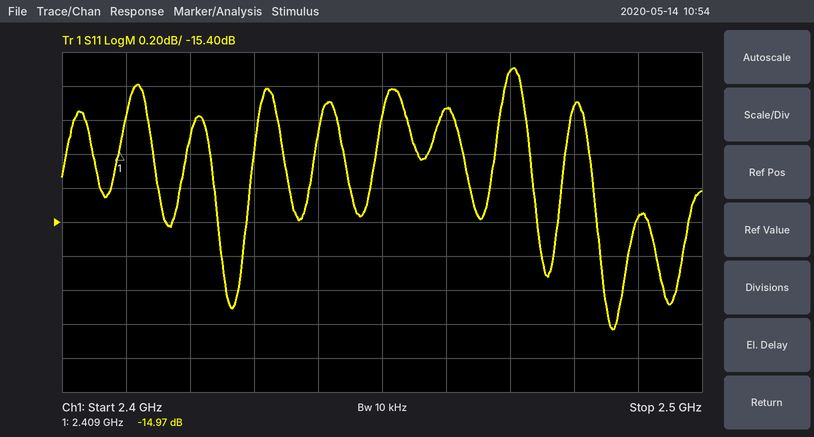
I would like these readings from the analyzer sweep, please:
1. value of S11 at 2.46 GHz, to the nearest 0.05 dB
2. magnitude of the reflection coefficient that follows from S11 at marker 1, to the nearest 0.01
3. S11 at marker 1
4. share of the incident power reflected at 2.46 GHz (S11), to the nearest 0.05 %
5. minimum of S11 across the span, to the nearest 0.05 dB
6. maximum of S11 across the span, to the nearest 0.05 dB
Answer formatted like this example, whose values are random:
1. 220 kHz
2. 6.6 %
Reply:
1. -14.75 dB
2. 0.18
3. -14.97 dB
4. 3.35 %
5. -16.05 dB
6. -14.50 dB
